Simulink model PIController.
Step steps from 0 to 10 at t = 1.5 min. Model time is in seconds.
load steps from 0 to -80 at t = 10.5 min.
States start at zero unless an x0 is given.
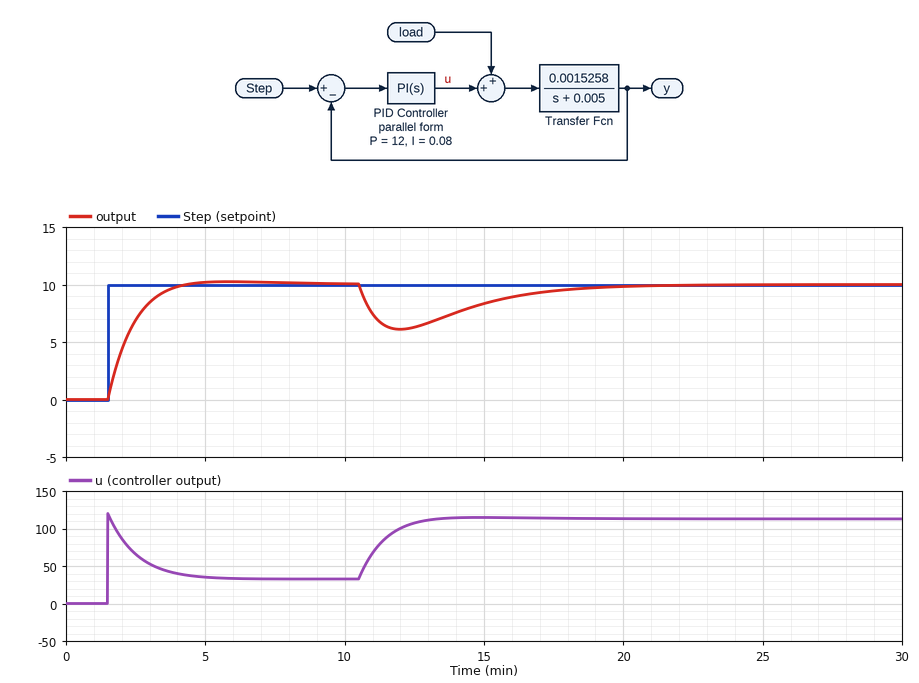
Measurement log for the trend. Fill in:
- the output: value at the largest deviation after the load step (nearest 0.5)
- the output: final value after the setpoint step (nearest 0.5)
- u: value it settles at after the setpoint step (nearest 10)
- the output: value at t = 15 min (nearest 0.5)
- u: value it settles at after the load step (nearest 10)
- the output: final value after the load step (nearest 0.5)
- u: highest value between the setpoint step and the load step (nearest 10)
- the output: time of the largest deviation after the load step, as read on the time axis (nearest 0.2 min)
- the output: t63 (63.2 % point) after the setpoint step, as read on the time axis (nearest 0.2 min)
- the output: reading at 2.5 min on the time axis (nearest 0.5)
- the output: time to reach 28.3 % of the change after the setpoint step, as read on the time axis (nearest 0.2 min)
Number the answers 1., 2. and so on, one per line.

1. 6.0
2. 10.0
3. 30
4. 8.5
5. 110
6. 10.0
7. 120
8. 12.0 min
9. 2.4 min
10. 7.0
11. 1.8 min
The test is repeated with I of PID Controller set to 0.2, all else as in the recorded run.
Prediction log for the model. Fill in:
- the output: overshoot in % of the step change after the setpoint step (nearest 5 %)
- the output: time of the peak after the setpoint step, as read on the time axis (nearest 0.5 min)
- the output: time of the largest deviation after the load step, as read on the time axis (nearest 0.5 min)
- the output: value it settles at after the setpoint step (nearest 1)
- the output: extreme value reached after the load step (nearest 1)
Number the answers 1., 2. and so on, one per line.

1. 15 %
2. 4.0 min
3. 11.5 min
4. 10
5. 7
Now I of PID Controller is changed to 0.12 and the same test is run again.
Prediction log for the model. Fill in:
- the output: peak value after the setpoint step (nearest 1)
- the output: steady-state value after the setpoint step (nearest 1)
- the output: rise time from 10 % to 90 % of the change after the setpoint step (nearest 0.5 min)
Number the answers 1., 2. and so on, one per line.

1. 11
2. 10
3. 1.5 min
